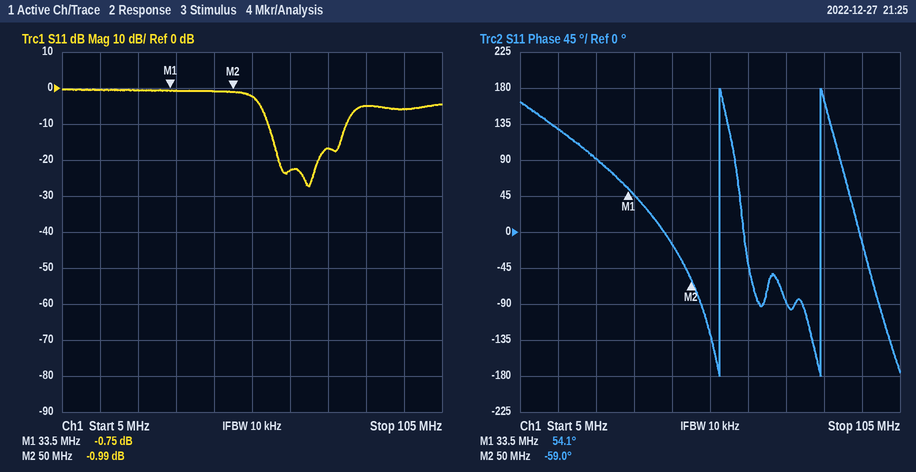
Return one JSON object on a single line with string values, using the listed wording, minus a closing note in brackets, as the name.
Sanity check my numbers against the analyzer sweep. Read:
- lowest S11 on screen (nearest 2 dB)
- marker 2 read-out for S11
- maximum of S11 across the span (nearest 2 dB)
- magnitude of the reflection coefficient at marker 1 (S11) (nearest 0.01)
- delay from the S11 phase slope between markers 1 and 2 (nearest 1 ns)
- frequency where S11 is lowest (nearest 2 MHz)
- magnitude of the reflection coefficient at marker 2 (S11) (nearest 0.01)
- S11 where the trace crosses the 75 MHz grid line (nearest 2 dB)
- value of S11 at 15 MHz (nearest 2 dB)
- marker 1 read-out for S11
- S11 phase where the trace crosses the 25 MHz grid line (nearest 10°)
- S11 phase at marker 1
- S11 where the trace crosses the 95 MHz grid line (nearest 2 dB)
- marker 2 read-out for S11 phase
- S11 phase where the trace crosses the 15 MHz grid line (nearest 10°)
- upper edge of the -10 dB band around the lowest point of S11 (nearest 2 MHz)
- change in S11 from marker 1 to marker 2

{"lowest S11 on screen": "-28 dB", "marker 2 read-out for S11": "-0.99 dB", "maximum of S11 across the span": "0 dB", "magnitude of the reflection coefficient at marker 1 (S11)": "0.92", "delay from the S11 phase slope between markers 1 and 2": "19 ns", "frequency where S11 is lowest": "70 MHz", "magnitude of the reflection coefficient at marker 2 (S11)": "0.89", "S11 where the trace crosses the 75 MHz grid line": "-16 dB", "value of S11 at 15 MHz": "0 dB", "marker 1 read-out for S11": "-0.75 dB", "S11 phase where the trace crosses the 25 MHz grid line": "90°", "S11 phase at marker 1": "54.1°", "S11 where the trace crosses the 95 MHz grid line": "-6 dB", "marker 2 read-out for S11 phase": "-59.0°", "S11 phase where the trace crosses the 15 MHz grid line": "130°", "upper edge of the -10 dB band around the lowest point of S11": "80 MHz", "change in S11 from marker 1 to marker 2": "-0.24 dB"}
